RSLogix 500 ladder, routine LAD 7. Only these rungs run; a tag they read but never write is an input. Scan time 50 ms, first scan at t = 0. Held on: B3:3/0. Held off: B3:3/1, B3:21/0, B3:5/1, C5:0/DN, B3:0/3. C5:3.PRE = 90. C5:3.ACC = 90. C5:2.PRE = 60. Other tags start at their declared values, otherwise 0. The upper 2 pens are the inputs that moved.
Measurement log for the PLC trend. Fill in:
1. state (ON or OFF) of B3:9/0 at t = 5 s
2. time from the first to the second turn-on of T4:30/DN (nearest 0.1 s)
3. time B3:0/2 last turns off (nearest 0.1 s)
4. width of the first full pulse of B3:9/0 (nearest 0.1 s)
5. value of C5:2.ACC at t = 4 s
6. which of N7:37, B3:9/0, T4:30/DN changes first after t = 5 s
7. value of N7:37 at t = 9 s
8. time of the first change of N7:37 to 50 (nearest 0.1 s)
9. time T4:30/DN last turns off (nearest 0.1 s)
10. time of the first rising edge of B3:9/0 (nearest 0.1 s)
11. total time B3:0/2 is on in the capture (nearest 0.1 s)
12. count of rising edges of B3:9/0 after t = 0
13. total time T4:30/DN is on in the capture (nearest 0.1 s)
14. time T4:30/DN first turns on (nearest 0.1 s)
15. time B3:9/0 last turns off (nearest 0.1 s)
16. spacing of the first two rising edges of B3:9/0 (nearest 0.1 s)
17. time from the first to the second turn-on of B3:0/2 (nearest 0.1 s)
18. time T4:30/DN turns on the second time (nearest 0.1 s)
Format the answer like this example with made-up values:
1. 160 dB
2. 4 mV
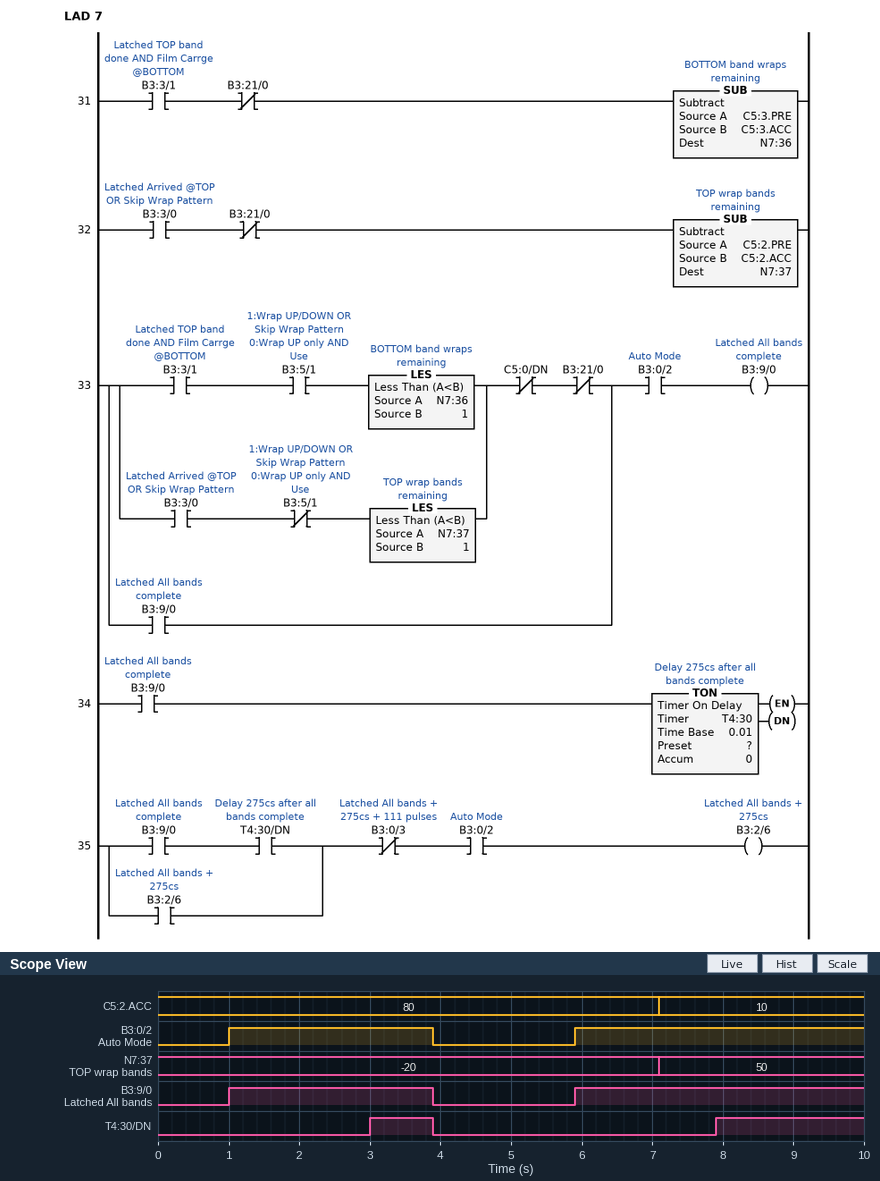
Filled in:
1. OFF
2. 4.9 s
3. 3.9 s
4. 2.9 s
5. 80
6. B3:9/0
7. 50
8. 7.1 s
9. 3.9 s
10. 1.0 s
11. 7.0 s
12. 2
13. 3.0 s
14. 3.0 s
15. 3.9 s
16. 4.9 s
17. 4.9 s
18. 7.9 s
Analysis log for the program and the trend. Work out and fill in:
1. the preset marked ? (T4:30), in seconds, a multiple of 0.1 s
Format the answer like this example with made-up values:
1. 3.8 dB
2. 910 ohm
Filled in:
1. 2.0 s
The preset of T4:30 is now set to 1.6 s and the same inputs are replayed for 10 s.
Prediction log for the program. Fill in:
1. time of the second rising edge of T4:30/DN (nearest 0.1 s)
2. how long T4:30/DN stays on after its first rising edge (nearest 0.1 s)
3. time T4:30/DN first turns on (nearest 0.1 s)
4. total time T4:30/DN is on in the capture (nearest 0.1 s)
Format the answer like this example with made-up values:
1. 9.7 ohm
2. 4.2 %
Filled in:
1. 7.5 s
2. 1.3 s
3. 2.6 s
4. 3.8 s
